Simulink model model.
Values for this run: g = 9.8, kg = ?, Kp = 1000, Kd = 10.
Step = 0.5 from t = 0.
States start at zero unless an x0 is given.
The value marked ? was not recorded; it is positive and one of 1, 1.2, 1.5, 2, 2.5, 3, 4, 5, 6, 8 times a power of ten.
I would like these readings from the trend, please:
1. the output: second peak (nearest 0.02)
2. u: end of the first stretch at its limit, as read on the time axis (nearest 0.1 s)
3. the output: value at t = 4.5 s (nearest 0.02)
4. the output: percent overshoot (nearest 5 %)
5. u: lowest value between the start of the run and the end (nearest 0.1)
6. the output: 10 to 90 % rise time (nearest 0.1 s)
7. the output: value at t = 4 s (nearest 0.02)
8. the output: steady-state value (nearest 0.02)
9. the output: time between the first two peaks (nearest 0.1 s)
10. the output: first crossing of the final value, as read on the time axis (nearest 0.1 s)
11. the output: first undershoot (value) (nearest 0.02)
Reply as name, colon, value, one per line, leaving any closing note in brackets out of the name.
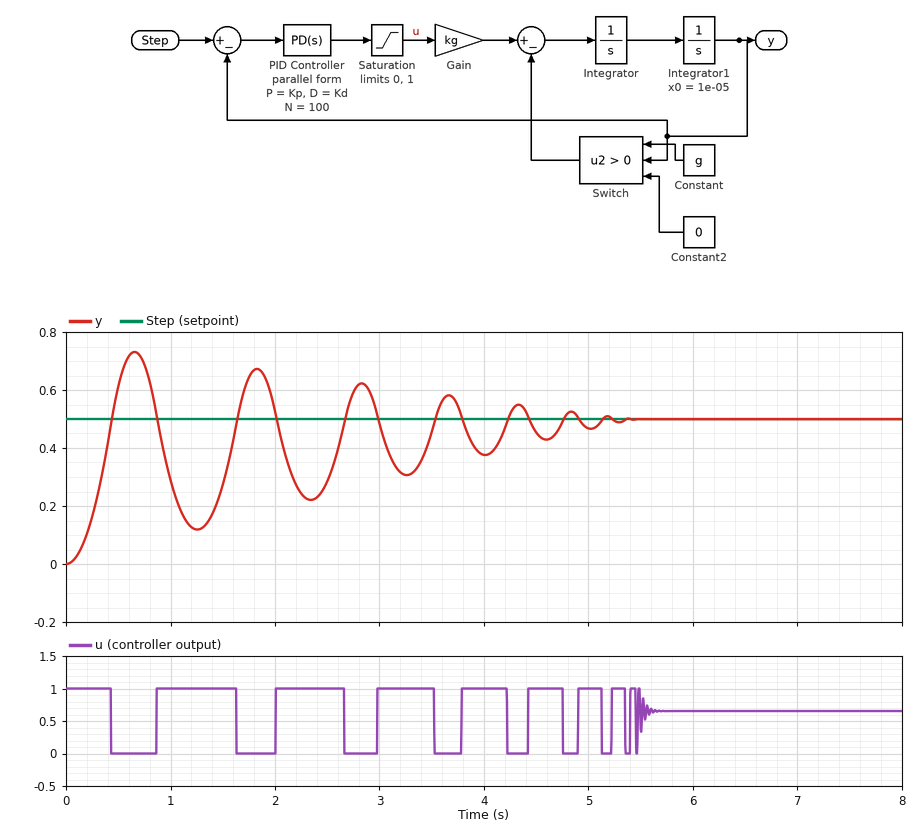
the output: second peak: 0.68
u: end of the first stretch at its limit, as read on the time axis: 0.4 s
the output: value at t = 4.5 s: 0.46
the output: percent overshoot: 45 %
u: lowest value between the start of the run and the end: 0.0
the output: 10 to 90 % rise time: 0.3 s
the output: value at t = 4 s: 0.38
the output: steady-state value: 0.50
the output: time between the first two peaks: 1.2 s
the output: first crossing of the final value, as read on the time axis: 0.4 s
the output: first undershoot (value): 0.12
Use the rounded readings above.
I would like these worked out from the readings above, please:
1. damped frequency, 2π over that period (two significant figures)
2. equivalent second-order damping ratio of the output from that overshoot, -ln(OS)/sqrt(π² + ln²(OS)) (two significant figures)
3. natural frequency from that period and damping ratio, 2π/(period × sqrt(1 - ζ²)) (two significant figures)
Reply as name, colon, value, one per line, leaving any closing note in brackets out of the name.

damped frequency, 2π over that period: 5.2 rad/s
equivalent second-order damping ratio of the output from that overshoot, -ln(OS)/sqrt(π² + ln²(OS)): 0.25
natural frequency from that period and damping ratio, 2π/(period × sqrt(1 - ζ²)): 5.4 rad/s
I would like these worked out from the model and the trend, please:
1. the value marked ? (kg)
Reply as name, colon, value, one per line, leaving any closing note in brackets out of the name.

the value marked ?: 15
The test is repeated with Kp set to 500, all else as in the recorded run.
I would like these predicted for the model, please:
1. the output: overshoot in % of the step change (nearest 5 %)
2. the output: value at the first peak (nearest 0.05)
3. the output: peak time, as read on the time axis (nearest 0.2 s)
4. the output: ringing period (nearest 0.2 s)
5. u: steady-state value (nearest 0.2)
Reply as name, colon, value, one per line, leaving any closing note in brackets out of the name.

the output: overshoot in % of the step change: 40 %
the output: value at the first peak: 0.70
the output: peak time, as read on the time axis: 0.6 s
the output: ringing period: 1.0 s
u: steady-state value: 0.6
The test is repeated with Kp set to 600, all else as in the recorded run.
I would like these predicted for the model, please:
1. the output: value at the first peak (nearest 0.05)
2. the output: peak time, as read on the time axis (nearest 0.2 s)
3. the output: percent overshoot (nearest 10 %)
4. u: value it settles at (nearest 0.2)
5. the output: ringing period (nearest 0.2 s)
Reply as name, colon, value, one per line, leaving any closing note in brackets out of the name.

the output: value at the first peak: 0.70
the output: peak time, as read on the time axis: 0.6 s
the output: percent overshoot: 40 %
u: value it settles at: 0.6
the output: ringing period: 1.0 s
